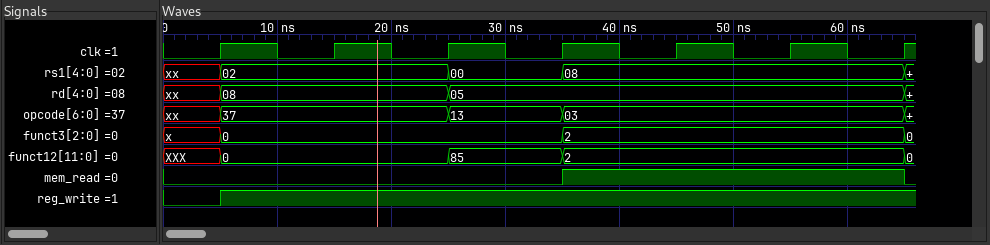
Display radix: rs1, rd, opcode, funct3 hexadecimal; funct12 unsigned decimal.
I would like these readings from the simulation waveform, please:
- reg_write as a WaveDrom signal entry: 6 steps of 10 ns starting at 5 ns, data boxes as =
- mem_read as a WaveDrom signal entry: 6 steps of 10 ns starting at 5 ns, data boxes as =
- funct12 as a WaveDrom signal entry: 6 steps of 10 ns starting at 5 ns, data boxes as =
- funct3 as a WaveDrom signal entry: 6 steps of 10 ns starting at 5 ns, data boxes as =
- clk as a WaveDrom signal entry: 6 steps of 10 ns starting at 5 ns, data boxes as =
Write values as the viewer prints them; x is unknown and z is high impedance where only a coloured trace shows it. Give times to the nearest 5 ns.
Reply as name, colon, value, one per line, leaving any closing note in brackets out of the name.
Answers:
reg_write as a WaveDrom signal entry: 6 steps of 10 ns starting at 5 ns, data boxes as =: {name: 'reg_write', wave: '1.....'}
mem_read as a WaveDrom signal entry: 6 steps of 10 ns starting at 5 ns, data boxes as =: {name: 'mem_read', wave: '0..1..'}
funct12 as a WaveDrom signal entry: 6 steps of 10 ns starting at 5 ns, data boxes as =: {name: 'funct12', wave: '=.==..', data: '0 85 2'}
funct3 as a WaveDrom signal entry: 6 steps of 10 ns starting at 5 ns, data boxes as =: {name: 'funct3', wave: '=..=..', data: '0 2'}
clk as a WaveDrom signal entry: 6 steps of 10 ns starting at 5 ns, data boxes as =: {name: 'clk', wave: 'p.....'}
